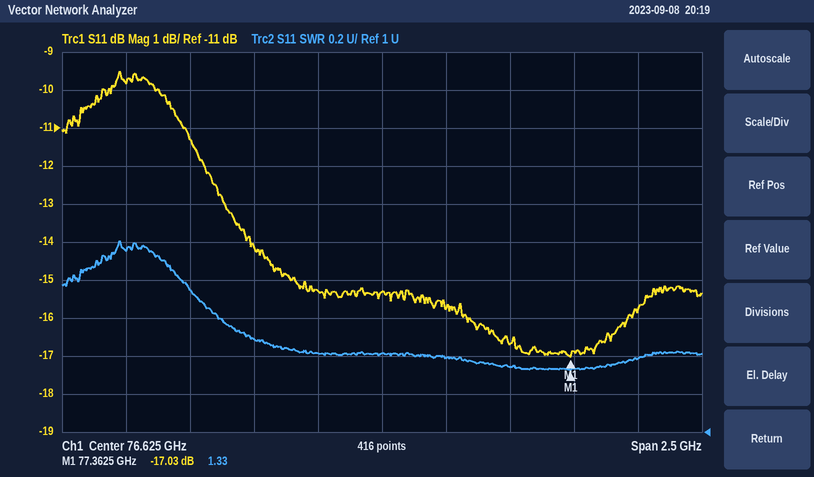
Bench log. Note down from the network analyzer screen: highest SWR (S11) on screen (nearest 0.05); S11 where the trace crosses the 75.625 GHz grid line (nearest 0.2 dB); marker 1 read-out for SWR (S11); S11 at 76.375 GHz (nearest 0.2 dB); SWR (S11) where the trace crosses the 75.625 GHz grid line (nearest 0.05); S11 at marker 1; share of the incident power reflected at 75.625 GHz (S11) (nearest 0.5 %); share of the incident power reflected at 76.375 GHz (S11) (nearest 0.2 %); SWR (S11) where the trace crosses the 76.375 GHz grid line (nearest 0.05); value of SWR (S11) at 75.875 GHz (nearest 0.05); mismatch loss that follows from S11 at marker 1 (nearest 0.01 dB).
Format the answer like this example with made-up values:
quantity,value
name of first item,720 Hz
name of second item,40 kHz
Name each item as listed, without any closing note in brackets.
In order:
quantity,value
highest SWR (S11) on screen,2.00
S11 where the trace crosses the 75.625 GHz grid line,-9.8 dB
marker 1 read-out for SWR,1.33
S11 at 76.375 GHz,-15.2 dB
SWR (S11) where the trace crosses the 75.625 GHz grid line,1.95
S11 at marker 1,-17.03 dB
share of the incident power reflected at 75.625 GHz (S11),10.5 %
share of the incident power reflected at 76.375 GHz (S11),3.0 %
SWR (S11) where the trace crosses the 76.375 GHz grid line,1.40
value of SWR (S11) at 75.875 GHz,1.75
mismatch loss that follows from S11 at marker 1,0.09 dB
